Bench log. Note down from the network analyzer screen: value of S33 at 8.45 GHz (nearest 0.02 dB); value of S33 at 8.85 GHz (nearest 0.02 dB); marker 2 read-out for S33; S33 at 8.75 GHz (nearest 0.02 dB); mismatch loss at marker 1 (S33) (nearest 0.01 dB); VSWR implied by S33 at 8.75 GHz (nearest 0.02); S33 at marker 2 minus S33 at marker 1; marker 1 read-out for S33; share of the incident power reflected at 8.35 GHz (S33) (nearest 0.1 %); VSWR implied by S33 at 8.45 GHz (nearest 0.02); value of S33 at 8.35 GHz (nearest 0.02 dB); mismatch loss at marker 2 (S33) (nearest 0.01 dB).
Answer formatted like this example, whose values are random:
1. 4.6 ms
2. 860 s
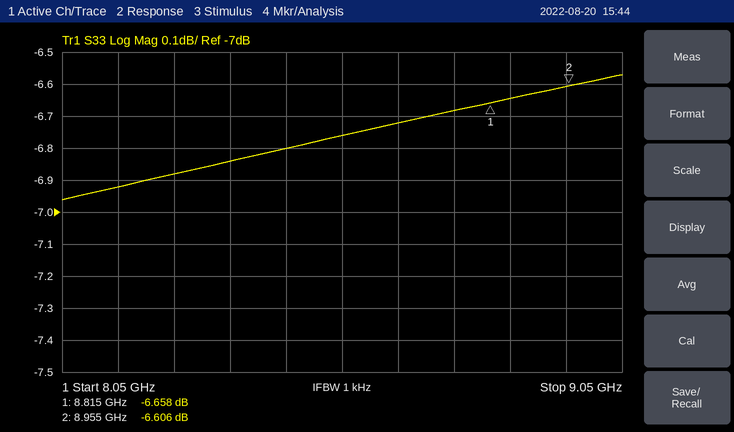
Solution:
1. -6.80 dB
2. -6.64 dB
3. -6.606 dB
4. -6.68 dB
5. 1.06 dB
6. 2.72
7. 0.052 dB
8. -6.658 dB
9. 20.7 %
10. 2.68
11. -6.84 dB
12. 1.07 dB
